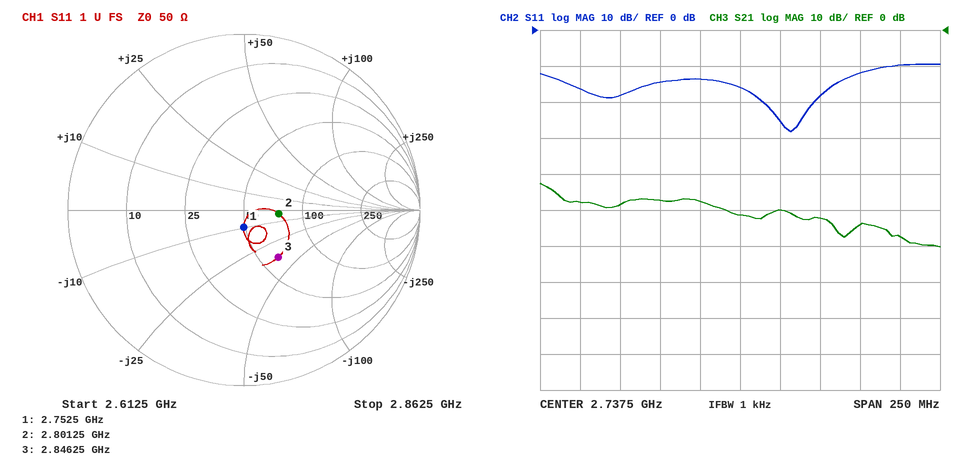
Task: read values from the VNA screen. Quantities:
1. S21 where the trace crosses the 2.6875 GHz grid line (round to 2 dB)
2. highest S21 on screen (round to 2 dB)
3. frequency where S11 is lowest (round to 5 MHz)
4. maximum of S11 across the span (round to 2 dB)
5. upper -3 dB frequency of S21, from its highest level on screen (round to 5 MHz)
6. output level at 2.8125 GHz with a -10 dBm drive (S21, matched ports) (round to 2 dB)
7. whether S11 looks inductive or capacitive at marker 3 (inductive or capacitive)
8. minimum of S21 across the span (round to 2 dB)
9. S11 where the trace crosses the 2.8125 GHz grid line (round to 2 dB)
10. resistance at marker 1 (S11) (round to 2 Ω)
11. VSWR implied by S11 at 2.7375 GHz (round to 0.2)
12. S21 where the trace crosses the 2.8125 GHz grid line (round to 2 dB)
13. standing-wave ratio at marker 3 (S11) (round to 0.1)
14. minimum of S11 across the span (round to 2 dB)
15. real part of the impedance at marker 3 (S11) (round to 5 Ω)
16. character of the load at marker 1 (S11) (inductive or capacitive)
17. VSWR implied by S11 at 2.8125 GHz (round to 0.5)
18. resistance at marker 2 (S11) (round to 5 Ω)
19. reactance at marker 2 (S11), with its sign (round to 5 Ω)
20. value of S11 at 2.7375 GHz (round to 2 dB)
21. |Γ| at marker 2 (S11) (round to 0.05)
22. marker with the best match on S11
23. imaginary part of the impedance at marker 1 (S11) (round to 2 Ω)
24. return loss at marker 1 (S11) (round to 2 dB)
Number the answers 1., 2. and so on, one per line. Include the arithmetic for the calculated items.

1. -48 dB
2. -42 dB
3. 2.770 GHz
4. -10 dB
5. 2.625 GHz
6. -10 dBm + (-54 dB) = -64 dBm
7. capacitive
8. -60 dB
9. -12 dB
10. 48 Ω
11. |Γ| = 10^(-16/20) = 0.1585; VSWR = (1 + 0.1585)/(1 − 0.1585) ≈ 1.4
12. -54 dB
13. 2.0
14. -28 dB
15. 60 Ω
16. capacitive
17. |Γ| = 10^(-12/20) = 0.2512; VSWR = (1 + 0.2512)/(1 − 0.2512) ≈ 1.67, so 1.5 to the nearest 0.5
18. 75 Ω
19. -5 Ω
20. -16 dB
21. 0.20
22. marker 1
23. -10 Ω
24. 20 dB
